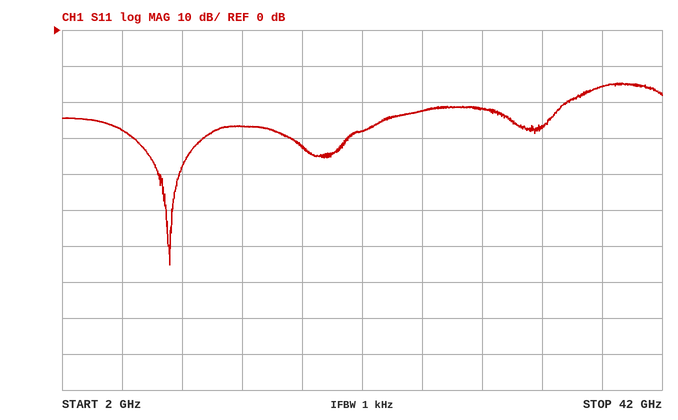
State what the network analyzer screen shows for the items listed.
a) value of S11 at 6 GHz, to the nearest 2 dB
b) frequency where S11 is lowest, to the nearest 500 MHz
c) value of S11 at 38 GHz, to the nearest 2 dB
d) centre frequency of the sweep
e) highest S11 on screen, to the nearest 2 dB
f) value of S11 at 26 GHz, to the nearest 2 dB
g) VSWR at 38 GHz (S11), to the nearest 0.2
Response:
-28 dB
9.0 GHz
-16 dB
22 GHz
-14 dB
-22 dB
1.4
